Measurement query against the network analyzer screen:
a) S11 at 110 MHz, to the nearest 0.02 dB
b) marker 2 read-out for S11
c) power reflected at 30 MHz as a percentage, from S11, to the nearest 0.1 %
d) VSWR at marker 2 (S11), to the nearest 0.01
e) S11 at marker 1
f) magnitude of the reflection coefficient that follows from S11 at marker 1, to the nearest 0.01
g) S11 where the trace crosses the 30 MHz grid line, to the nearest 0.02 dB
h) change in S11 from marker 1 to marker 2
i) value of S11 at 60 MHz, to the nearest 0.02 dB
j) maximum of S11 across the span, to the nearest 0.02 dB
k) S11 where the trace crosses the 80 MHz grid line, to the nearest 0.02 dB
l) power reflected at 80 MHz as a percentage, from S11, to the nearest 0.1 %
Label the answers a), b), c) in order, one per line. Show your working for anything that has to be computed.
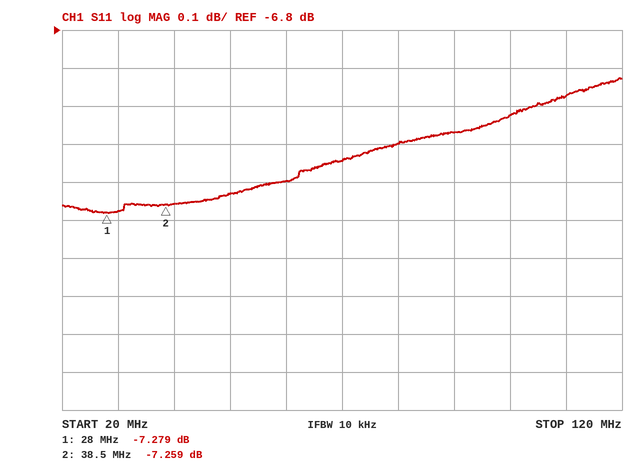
a) -6.98 dB
b) -7.259 dB
c) 10^(-7.28/10) ≈ 18.7 %
d) (1 + 0.4336)/(1 − 0.4336) ≈ 2.53
e) -7.279 dB
f) 10^(-7.279/20) ≈ 0.43
g) -7.28 dB
h) -7.259 − (-7.279) = 0.020 dB
i) -7.20 dB
j) -6.92 dB
k) -7.10 dB
l) 10^(-7.1/10) ≈ 19.5 %
